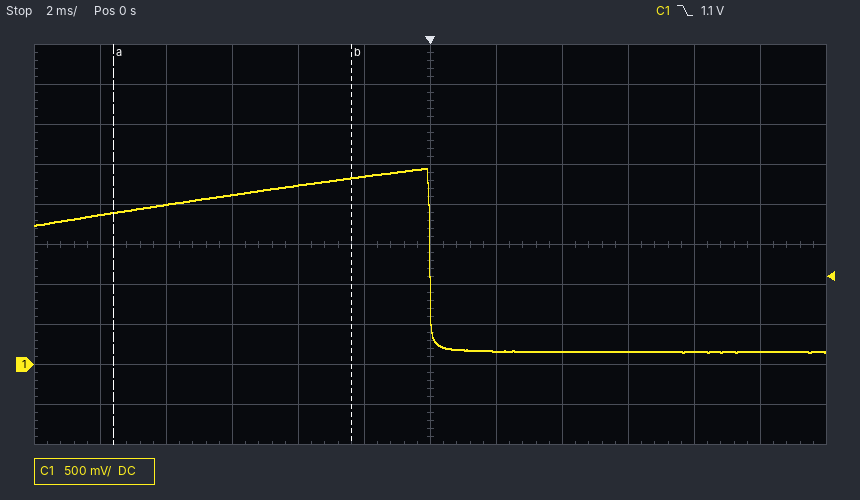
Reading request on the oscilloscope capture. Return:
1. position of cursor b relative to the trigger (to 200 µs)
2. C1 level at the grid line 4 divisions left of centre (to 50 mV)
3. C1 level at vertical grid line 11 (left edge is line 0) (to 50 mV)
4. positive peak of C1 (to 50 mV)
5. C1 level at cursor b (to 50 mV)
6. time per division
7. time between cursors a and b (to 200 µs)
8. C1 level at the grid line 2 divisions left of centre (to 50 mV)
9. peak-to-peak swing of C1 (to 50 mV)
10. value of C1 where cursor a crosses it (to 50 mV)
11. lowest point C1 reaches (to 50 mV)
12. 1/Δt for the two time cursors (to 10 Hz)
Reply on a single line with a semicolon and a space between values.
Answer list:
-2.4 ms; 2.00 V; 150 mV; 2.45 V; 2.35 V; 2 ms; 7.2 ms; 2.25 V; 2.30 V; 1.90 V; 150 mV; 140 Hz
